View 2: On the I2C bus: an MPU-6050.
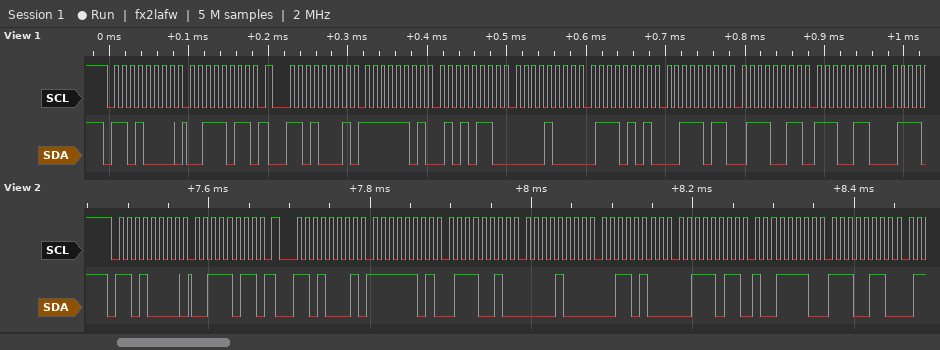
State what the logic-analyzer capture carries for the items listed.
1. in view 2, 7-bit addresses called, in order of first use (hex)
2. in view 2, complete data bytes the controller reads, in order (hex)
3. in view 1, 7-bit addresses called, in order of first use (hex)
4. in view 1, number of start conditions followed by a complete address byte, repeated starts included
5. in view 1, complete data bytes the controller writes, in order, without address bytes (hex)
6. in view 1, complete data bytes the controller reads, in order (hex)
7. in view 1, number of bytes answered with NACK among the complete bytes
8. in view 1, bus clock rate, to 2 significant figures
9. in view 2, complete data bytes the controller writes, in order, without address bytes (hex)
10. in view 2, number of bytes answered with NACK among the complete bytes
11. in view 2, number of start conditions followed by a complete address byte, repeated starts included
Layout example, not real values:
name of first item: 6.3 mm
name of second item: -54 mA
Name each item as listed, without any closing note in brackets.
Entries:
in view 2, 7-bit addresses called, in order of first use: 0x68
in view 2, complete data bytes the controller reads, in order: FD 72 08 34 3B 9E E6
in view 1, 7-bit addresses called, in order of first use: 0x68
in view 1, number of start conditions followed by a complete address byte, repeated starts included: 2
in view 1, complete data bytes the controller writes, in order, without address bytes: 3B
in view 1, complete data bytes the controller reads, in order: FD 56 08 75 3B 73 E6
in view 1, number of bytes answered with NACK among the complete bytes: 0
in view 1, bus clock rate, to 2 significant figures: 100 kHz
in view 2, complete data bytes the controller writes, in order, without address bytes: 3B
in view 2, number of bytes answered with NACK among the complete bytes: 0
in view 2, number of start conditions followed by a complete address byte, repeated starts included: 2
